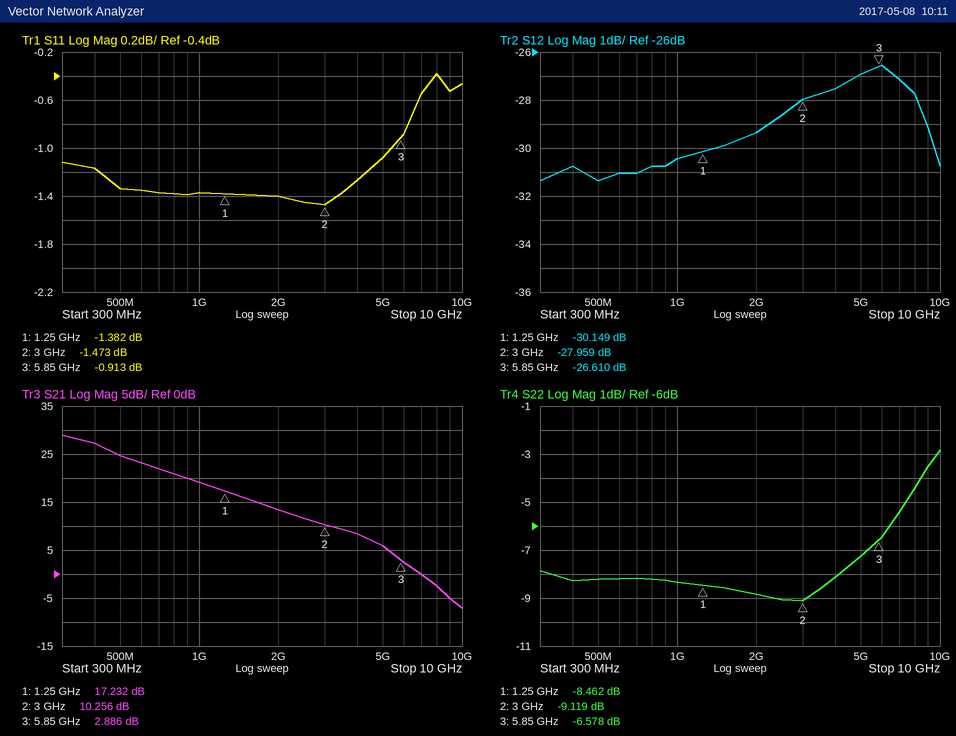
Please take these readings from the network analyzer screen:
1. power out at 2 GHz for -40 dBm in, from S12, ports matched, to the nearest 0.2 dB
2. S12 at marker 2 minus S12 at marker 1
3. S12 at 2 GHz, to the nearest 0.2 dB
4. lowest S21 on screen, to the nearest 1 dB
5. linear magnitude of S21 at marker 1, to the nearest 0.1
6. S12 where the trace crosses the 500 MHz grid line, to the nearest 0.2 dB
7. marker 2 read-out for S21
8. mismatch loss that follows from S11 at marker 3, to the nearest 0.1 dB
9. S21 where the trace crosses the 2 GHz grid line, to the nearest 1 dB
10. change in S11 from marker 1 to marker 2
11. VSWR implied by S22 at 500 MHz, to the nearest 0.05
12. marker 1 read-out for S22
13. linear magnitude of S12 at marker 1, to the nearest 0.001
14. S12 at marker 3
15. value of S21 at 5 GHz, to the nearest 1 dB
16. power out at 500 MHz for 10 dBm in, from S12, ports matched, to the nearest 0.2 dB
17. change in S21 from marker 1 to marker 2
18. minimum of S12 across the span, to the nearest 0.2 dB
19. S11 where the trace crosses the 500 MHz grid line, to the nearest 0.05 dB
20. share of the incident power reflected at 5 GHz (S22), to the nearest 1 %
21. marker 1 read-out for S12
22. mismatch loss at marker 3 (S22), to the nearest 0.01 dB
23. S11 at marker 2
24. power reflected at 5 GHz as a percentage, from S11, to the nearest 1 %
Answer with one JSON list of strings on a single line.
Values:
["-69.4 dBm", "2.190 dB", "-29.4 dB", "-7 dB", "7.3", "-31.4 dB", "10.256 dB", "7.2 dB", "13 dB", "-0.091 dB", "2.25", "-8.462 dB", "0.031", "-26.610 dB", "6 dB", "-21.4 dBm", "-6.976 dB", "-31.4 dB", "-1.35 dB", "19 %", "-30.149 dB", "1.08 dB", "-1.473 dB", "78 %"]
